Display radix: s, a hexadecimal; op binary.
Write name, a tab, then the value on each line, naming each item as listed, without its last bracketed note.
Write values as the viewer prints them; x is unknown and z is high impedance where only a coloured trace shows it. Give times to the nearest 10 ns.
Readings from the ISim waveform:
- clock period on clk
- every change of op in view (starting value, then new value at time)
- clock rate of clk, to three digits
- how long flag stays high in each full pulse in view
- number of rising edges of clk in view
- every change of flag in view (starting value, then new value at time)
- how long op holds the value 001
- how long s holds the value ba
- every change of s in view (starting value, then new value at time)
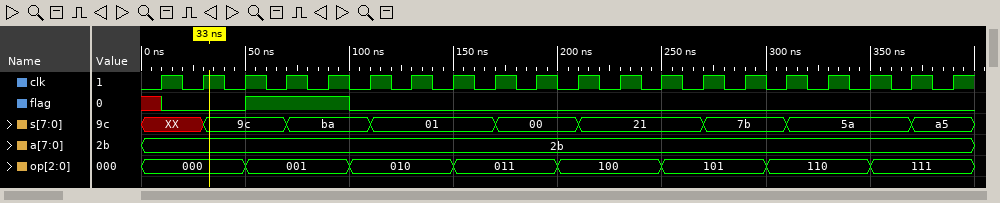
clock period on clk	20 ns
every change of op in view	000, 001 at 50 ns, 010 at 100 ns, 011 at 150 ns, 100 at 200 ns, 101 at 250 ns, 110 at 300 ns, 111 at 350 ns
clock rate of clk, to three digits	50.0 MHz
how long flag stays high in each full pulse in view	50 ns
number of rising edges of clk in view	20
every change of flag in view	x, 0 at 10 ns, 1 at 50 ns, 0 at 100 ns
how long op holds the value 001	50 ns
how long s holds the value ba	40 ns
every change of s in view	XX, 9c at 30 ns, ba at 70 ns, 01 at 110 ns, 00 at 170 ns, 21 at 210 ns, 7b at 270 ns, 5a at 310 ns, a5 at 370 ns
